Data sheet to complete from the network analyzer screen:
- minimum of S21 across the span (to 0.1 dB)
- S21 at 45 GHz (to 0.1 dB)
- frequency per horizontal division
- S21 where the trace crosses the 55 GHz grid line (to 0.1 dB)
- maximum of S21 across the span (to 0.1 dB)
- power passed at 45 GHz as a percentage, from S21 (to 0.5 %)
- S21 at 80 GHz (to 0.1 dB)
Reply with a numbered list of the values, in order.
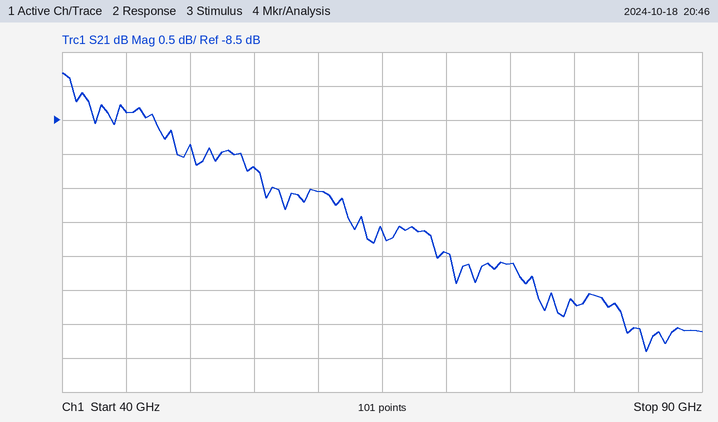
1. -11.9 dB
2. -8.4 dB
3. 5 GHz
4. -9.2 dB
5. -7.8 dB
6. 14.5 %
7. -11.2 dB
